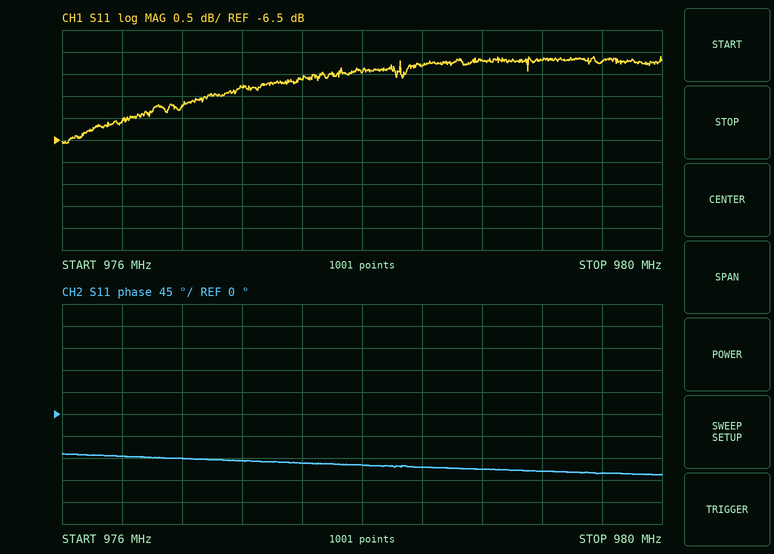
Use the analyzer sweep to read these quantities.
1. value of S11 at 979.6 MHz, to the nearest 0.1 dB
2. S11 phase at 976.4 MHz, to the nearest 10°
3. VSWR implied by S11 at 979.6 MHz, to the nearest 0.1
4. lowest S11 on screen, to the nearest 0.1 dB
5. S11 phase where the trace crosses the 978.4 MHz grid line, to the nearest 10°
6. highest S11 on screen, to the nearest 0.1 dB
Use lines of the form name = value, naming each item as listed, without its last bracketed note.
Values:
value of S11 at 979.6 MHz, to the nearest 0.1 dB = -4.7 dB
S11 phase at 976.4 MHz, to the nearest 10° = -90°
VSWR implied by S11 at 979.6 MHz, to the nearest 0.1 = 3.8
lowest S11 on screen, to the nearest 0.1 dB = -6.6 dB
S11 phase where the trace crosses the 978.4 MHz grid line, to the nearest 10° = -110°
highest S11 on screen, to the nearest 0.1 dB = -4.6 dB
